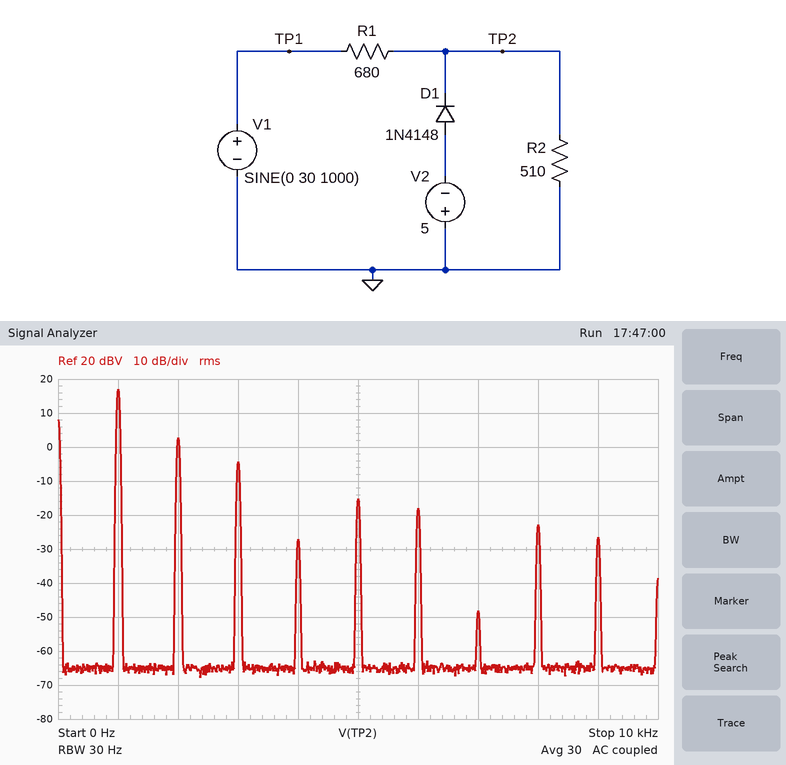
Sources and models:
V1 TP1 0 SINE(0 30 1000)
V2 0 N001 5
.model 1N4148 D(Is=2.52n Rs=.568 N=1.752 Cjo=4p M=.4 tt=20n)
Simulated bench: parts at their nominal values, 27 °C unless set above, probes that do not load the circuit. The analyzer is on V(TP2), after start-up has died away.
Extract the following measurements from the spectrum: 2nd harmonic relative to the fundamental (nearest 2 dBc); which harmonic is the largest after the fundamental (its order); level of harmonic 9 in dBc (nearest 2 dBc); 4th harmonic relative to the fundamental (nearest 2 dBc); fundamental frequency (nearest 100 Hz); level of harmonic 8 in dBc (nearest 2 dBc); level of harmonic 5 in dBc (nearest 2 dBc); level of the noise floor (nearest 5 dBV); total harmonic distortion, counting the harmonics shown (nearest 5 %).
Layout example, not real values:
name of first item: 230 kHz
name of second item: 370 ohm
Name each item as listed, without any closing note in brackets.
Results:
2nd harmonic relative to the fundamental: -14 dBc
which harmonic is the largest after the fundamental: 2
level of harmonic 9 in dBc: -44 dBc
4th harmonic relative to the fundamental: -44 dBc
fundamental frequency: 1.0 kHz
level of harmonic 8 in dBc: -40 dBc
level of harmonic 5 in dBc: -32 dBc
level of the noise floor: -65 dBV
total harmonic distortion, counting the harmonics shown: 20 %
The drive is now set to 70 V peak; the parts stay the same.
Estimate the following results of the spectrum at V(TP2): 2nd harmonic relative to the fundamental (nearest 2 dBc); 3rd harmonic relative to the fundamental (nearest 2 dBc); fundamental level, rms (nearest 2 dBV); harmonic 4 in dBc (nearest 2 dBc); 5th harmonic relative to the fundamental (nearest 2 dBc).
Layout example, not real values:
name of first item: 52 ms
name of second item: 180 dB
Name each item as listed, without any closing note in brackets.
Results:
2nd harmonic relative to the fundamental: -10 dBc
3rd harmonic relative to the fundamental: -24 dBc
fundamental level, rms: 22 dBV
harmonic 4 in dBc: -26 dBc
5th harmonic relative to the fundamental: -30 dBc
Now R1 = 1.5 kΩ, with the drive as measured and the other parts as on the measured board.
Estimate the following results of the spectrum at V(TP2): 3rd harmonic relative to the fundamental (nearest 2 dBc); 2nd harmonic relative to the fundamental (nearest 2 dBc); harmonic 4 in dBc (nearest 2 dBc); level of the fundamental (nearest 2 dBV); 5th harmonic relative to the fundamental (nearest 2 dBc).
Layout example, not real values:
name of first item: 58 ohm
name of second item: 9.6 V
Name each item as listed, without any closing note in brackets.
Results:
3rd harmonic relative to the fundamental: -26 dBc
2nd harmonic relative to the fundamental: -24 dBc
harmonic 4 in dBc: -30 dBc
level of the fundamental: 14 dBV
5th harmonic relative to the fundamental: -38 dBc
